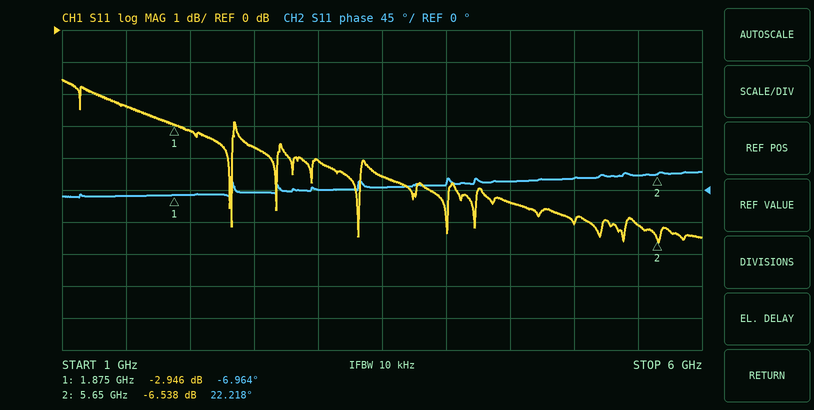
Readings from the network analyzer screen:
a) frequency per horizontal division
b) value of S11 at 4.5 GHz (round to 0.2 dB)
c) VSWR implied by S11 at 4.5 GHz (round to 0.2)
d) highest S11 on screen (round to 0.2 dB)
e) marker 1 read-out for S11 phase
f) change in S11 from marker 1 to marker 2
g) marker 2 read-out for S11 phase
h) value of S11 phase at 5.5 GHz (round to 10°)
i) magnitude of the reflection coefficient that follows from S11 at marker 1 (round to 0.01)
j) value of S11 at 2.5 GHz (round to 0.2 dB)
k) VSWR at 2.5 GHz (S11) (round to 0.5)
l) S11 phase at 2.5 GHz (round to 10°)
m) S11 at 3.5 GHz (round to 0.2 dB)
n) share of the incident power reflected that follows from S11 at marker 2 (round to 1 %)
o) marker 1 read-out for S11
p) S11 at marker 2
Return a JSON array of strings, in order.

["500 MHz", "-5.4 dB", "3.4", "-1.6 dB", "-6.964°", "-3.592 dB", "22.218°", "20°", "0.71", "-3.6 dB", "5.0", "0°", "-4.6 dB", "22 %", "-2.946 dB", "-6.538 dB"]
